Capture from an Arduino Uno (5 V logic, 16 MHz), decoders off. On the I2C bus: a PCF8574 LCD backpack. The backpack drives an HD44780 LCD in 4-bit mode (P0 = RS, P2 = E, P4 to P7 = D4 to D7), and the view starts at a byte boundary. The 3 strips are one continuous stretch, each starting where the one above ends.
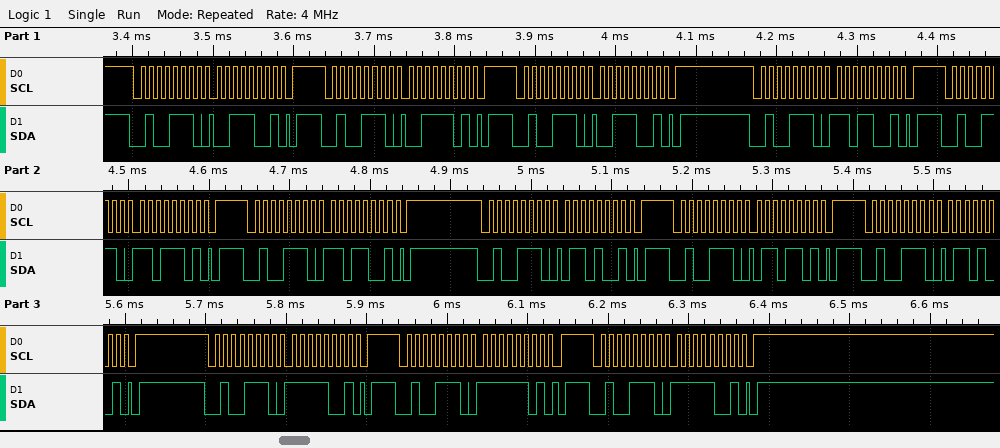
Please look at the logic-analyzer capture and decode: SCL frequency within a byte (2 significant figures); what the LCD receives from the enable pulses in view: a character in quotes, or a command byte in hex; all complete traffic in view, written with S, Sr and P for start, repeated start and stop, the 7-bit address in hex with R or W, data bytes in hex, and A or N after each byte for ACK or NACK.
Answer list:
100 kHz
'=' 'o'
S 27W A 39 A P S 27W A 3D A P S 27W A 39 A P S 27W A D9 A P S 27W A DD A P S 27W A D9 A P S 27W A 69 A P S 27W A 6D A P S 27W A 69 A P S 27W A F9 A P S 27W A FD A P S 27W A F9 A P
